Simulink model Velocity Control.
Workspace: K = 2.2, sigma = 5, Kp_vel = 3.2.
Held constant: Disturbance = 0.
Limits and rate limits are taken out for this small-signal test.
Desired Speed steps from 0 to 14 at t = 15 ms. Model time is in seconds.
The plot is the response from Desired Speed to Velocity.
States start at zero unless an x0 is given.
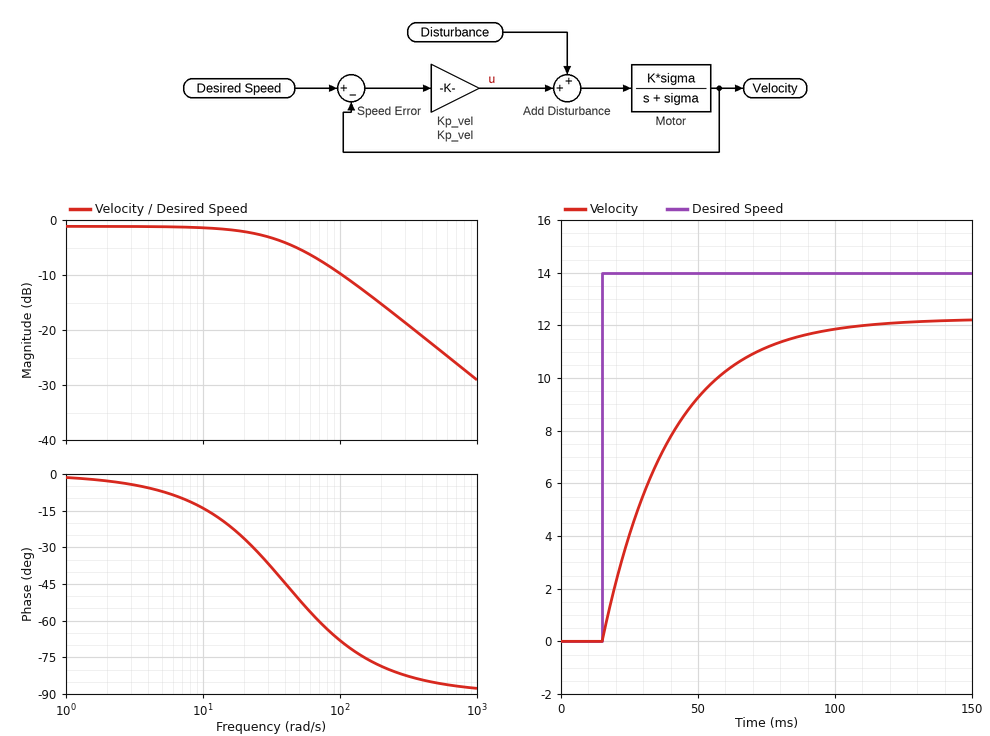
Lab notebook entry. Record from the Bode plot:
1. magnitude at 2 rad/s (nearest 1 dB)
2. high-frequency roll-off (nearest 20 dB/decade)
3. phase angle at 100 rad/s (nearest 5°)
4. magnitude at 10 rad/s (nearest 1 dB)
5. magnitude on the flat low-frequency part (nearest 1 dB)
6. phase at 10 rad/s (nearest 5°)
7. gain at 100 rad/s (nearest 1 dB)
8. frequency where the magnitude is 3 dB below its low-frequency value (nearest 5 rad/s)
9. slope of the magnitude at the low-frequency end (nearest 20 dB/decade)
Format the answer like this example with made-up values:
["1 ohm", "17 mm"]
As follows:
["-1 dB", "-20 dB/decade", "-70°", "-1 dB", "-1 dB", "-15°", "-10 dB", "40 rad/s", "0 dB/decade"]
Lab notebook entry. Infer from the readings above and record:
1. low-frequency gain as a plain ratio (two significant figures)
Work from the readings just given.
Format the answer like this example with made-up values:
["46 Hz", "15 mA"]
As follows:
["0.89"]
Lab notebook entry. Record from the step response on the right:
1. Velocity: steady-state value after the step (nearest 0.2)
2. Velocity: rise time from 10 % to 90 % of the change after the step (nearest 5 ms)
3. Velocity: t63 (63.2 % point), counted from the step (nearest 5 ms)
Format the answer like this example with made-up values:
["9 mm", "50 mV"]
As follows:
["12.2", "55 ms", "25 ms"]
